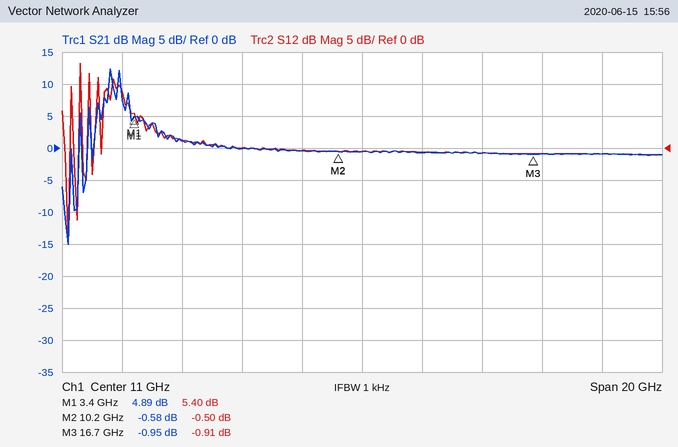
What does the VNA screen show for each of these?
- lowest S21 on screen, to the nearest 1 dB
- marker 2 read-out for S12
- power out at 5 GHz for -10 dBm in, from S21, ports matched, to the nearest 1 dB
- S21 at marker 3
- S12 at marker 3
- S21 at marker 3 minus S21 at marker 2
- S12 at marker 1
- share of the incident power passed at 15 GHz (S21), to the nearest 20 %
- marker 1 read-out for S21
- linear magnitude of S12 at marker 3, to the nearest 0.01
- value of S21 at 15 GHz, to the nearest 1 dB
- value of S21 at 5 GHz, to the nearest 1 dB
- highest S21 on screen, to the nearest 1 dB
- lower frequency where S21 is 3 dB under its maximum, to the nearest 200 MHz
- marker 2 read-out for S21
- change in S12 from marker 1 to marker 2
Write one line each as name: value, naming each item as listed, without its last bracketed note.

lowest S21 on screen, to the nearest 1 dB: -15 dB
marker 2 read-out for S12: -0.50 dB
power out at 5 GHz for -10 dBm in, from S21, ports matched, to the nearest 1 dB: -9 dBm
S21 at marker 3: -0.95 dB
S12 at marker 3: -0.91 dB
S21 at marker 3 minus S21 at marker 2: -0.37 dB
S12 at marker 1: 5.40 dB
share of the incident power passed at 15 GHz (S21), to the nearest 20 %: 80 %
marker 1 read-out for S21: 4.89 dB
linear magnitude of S12 at marker 3, to the nearest 0.01: 0.90
value of S21 at 15 GHz, to the nearest 1 dB: -1 dB
value of S21 at 5 GHz, to the nearest 1 dB: 1 dB
highest S21 on screen, to the nearest 1 dB: 12 dB
lower frequency where S21 is 3 dB under its maximum, to the nearest 200 MHz: 2.6 GHz
marker 2 read-out for S21: -0.58 dB
change in S12 from marker 1 to marker 2: -5.90 dB
